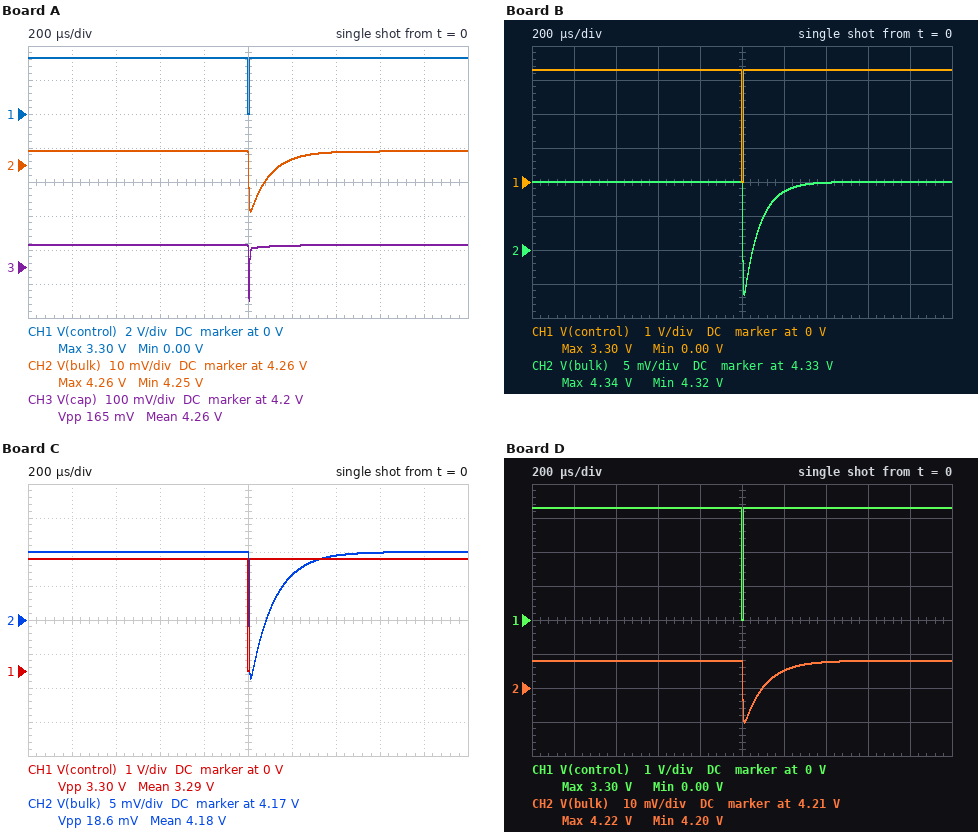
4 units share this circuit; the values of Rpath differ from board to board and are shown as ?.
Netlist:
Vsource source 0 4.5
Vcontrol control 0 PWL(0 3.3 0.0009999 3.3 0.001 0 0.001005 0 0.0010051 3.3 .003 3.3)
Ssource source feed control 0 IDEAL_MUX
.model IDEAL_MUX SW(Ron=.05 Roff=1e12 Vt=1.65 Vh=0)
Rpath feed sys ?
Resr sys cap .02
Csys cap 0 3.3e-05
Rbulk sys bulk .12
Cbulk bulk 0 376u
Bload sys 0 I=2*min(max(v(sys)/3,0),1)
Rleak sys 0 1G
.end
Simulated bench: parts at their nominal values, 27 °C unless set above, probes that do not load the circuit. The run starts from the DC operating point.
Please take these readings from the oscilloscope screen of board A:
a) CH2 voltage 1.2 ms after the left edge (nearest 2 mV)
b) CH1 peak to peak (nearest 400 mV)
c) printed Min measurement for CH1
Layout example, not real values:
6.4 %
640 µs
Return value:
4.262 V
3.2 V
0.00 V
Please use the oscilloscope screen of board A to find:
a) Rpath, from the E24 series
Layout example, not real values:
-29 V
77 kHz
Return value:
0.068 Ω
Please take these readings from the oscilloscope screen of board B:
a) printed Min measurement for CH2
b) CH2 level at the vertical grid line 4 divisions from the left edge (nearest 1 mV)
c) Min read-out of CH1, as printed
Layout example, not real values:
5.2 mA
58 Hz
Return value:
4.32 V
4.340 V
0.00 V
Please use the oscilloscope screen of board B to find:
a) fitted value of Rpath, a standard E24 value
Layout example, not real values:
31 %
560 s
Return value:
0.03 Ω
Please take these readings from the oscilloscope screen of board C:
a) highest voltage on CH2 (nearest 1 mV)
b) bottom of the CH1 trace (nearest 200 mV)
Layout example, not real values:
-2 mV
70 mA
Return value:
4.180 V
0 V
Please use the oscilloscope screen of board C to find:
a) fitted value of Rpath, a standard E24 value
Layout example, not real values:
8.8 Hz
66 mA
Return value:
0.11 Ω
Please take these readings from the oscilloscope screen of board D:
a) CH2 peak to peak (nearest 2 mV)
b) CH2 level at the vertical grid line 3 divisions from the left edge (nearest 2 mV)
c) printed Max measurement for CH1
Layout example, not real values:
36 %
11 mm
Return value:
18 mV
4.218 V
3.30 V
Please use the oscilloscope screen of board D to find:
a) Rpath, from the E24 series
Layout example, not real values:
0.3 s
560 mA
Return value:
0.091 Ω
